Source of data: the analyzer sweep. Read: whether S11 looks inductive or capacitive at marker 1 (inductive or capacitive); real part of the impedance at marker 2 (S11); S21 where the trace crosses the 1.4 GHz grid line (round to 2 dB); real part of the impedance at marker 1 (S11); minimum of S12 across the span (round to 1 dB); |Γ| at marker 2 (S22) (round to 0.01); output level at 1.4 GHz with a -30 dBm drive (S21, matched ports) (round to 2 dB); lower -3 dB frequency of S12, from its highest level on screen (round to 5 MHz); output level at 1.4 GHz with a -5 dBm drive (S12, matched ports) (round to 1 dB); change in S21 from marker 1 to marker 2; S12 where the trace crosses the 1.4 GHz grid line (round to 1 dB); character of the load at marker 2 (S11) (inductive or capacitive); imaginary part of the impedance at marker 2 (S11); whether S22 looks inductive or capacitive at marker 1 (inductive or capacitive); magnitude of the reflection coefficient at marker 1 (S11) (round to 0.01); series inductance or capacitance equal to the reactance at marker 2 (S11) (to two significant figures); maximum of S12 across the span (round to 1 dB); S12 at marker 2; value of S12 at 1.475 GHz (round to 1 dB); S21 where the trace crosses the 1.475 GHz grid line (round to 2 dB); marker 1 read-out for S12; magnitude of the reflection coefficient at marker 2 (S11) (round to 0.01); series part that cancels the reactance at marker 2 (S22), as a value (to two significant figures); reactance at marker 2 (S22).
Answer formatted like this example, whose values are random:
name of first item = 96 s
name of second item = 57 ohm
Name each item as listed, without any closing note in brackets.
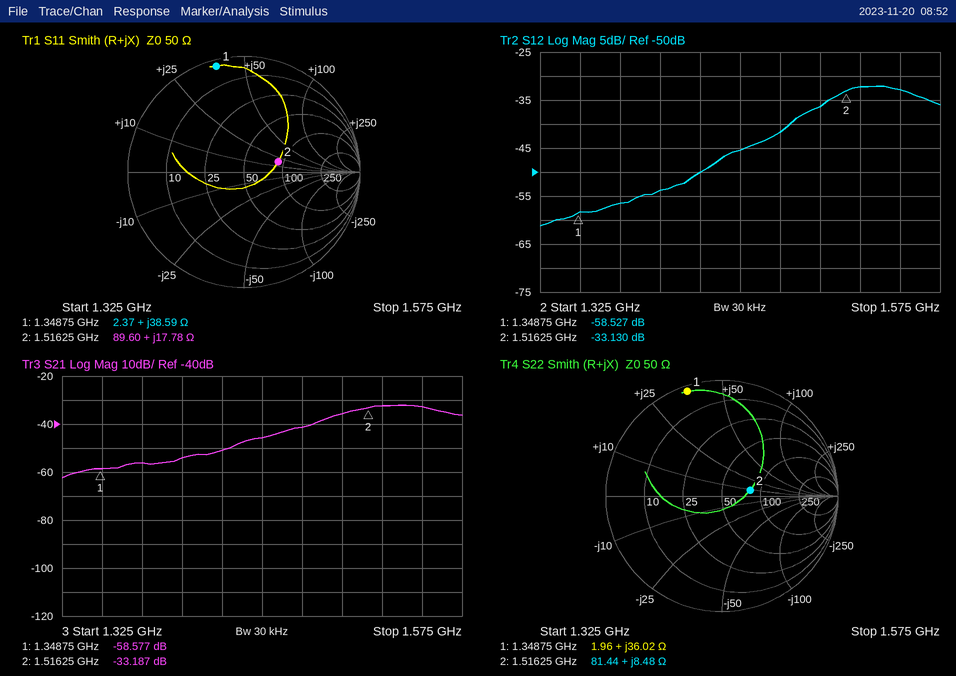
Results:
whether S11 looks inductive or capacitive at marker 1 = inductive
real part of the impedance at marker 2 = 89.60 Ω
S21 where the trace crosses the 1.4 GHz grid line = -54 dB
real part of the impedance at marker 1 = 2.37 Ω
minimum of S12 across the span = -61 dB
|Γ| at marker 2 (S22) = 0.25
output level at 1.4 GHz with a -30 dBm drive (S21, matched ports) = -84 dBm
lower -3 dB frequency of S12, from its highest level on screen = 1.505 GHz
output level at 1.4 GHz with a -5 dBm drive (S12, matched ports) = -59 dBm
change in S21 from marker 1 to marker 2 = 25.390 dB
S12 where the trace crosses the 1.4 GHz grid line = -54 dB
character of the load at marker 2 (S11) = inductive
imaginary part of the impedance at marker 2 = +17.78 Ω
whether S22 looks inductive or capacitive at marker 1 = inductive
magnitude of the reflection coefficient at marker 1 (S11) = 0.94
series inductance or capacitance equal to the reactance at marker 2 (S11) = 1.9 nH
maximum of S12 across the span = -32 dB
S12 at marker 2 = -33.130 dB
value of S12 at 1.475 GHz = -42 dB
S21 where the trace crosses the 1.475 GHz grid line = -42 dB
marker 1 read-out for S12 = -58.527 dB
magnitude of the reflection coefficient at marker 2 (S11) = 0.31
series part that cancels the reactance at marker 2 (S22), as a value = 12 pF
reactance at marker 2 = +8.48 Ω
